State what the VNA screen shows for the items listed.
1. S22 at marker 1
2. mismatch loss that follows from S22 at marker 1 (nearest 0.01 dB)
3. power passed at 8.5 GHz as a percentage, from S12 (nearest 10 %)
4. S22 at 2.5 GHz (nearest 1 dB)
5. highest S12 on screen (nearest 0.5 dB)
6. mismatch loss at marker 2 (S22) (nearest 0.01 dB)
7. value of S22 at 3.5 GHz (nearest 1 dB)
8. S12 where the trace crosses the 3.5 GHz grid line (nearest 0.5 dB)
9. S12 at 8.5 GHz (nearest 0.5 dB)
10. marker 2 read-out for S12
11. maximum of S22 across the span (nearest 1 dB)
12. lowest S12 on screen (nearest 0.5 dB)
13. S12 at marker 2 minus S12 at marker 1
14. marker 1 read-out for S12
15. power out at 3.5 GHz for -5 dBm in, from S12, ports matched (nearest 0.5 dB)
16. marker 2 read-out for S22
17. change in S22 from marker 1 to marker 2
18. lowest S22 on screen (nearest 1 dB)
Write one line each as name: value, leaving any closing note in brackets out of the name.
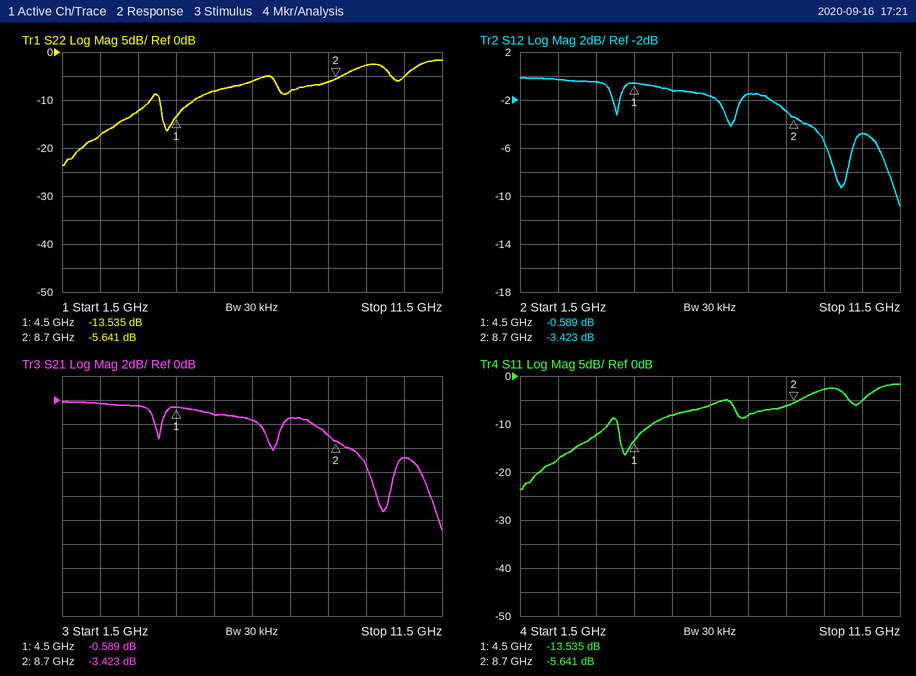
S22 at marker 1: -13.535 dB
mismatch loss that follows from S22 at marker 1: 0.20 dB
power passed at 8.5 GHz as a percentage, from S12: 50 %
S22 at 2.5 GHz: -17 dB
highest S12 on screen: 0.0 dB
mismatch loss at marker 2 (S22): 1.38 dB
value of S22 at 3.5 GHz: -12 dB
S12 where the trace crosses the 3.5 GHz grid line: -0.5 dB
S12 at 8.5 GHz: -3.0 dB
marker 2 read-out for S12: -3.423 dB
maximum of S22 across the span: -2 dB
lowest S12 on screen: -11.0 dB
S12 at marker 2 minus S12 at marker 1: -2.834 dB
marker 1 read-out for S12: -0.589 dB
power out at 3.5 GHz for -5 dBm in, from S12, ports matched: -5.5 dBm
marker 2 read-out for S22: -5.641 dB
change in S22 from marker 1 to marker 2: 7.894 dB
lowest S22 on screen: -24 dB
